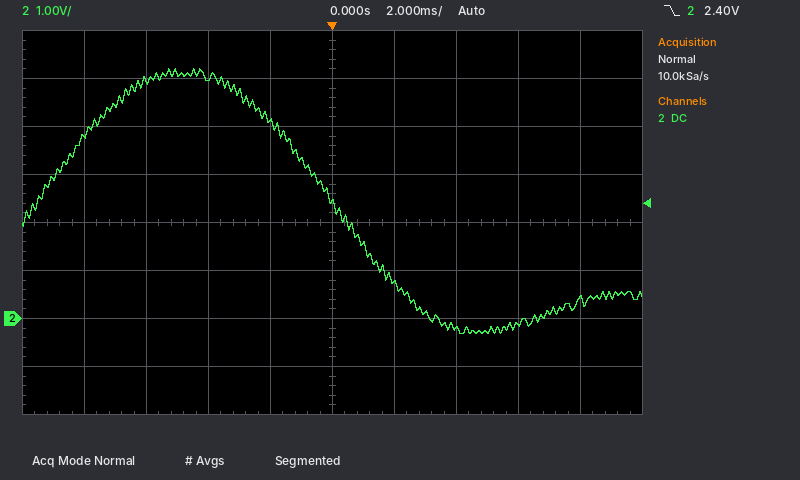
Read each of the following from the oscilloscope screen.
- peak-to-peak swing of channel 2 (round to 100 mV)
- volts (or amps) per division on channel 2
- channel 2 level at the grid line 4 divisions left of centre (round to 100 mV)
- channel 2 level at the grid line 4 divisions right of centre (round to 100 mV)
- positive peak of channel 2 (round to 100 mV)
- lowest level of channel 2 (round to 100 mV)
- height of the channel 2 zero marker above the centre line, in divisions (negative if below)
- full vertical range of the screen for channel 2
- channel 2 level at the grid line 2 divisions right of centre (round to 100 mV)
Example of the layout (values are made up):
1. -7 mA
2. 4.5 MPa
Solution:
1. 5.5 V
2. 1 V
3. 3.8 V
4. 400 mV
5. 5.2 V
6. -300 mV
7. -2.0 div
8. 8 V
9. -200 mV
